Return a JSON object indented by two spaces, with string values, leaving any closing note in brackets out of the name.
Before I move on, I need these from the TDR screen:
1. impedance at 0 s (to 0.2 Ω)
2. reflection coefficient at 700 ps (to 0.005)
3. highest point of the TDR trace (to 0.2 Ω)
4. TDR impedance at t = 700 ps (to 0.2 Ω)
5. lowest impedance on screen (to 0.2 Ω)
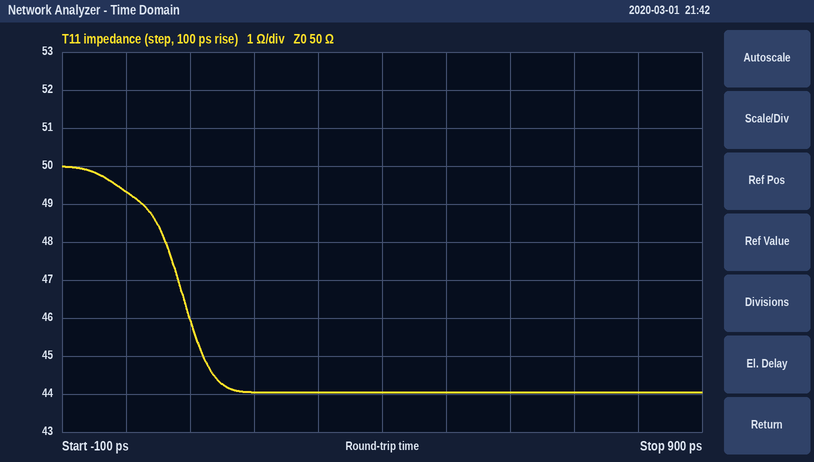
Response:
{
  "impedance at 0 s": "49.4 Ω",
  "reflection coefficient at 700 ps": "-0.065",
  "highest point of the TDR trace": "50.0 Ω",
  "TDR impedance at t = 700 ps": "44.0 Ω",
  "lowest impedance on screen": "44.0 Ω"
}
